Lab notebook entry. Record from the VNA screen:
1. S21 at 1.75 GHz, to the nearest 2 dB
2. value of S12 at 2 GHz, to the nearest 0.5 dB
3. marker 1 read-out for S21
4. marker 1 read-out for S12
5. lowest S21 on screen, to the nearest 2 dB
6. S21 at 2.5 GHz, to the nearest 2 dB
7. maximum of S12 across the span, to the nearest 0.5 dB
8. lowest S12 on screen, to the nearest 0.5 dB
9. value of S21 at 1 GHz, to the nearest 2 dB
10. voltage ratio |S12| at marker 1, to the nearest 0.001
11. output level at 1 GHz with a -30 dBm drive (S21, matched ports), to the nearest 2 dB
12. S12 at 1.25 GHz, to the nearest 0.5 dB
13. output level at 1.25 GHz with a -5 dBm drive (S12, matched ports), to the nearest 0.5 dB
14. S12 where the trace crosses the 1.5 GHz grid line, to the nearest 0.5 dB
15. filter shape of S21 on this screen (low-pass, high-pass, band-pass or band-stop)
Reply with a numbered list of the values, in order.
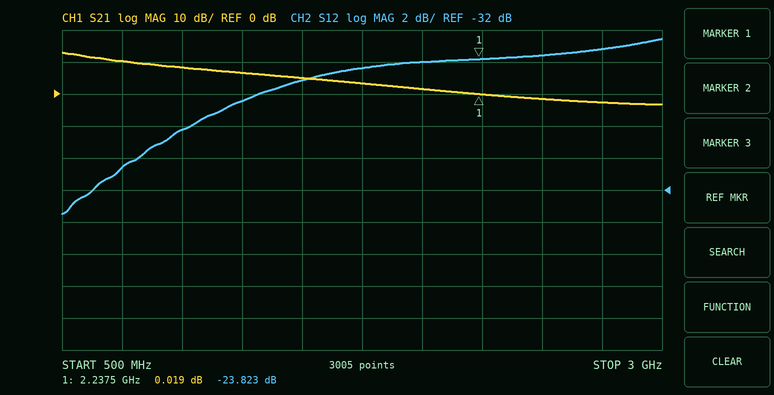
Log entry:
1. 4 dB
2. -24.0 dB
3. 0.019 dB
4. -23.823 dB
5. -4 dB
6. -2 dB
7. -22.5 dB
8. -33.5 dB
9. 8 dB
10. 0.064
11. -22 dBm
12. -26.5 dB
13. -31.5 dBm
14. -25.0 dB
15. low-pass
